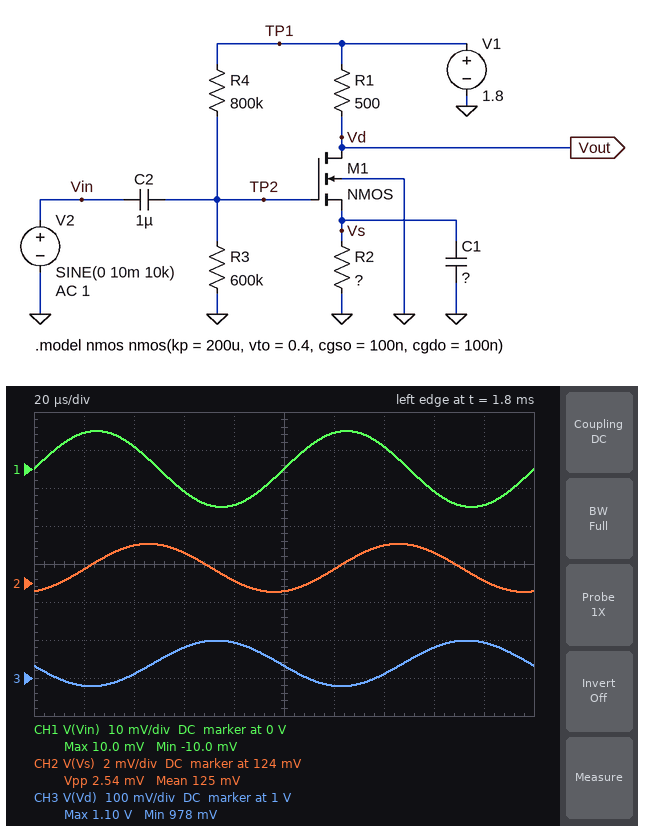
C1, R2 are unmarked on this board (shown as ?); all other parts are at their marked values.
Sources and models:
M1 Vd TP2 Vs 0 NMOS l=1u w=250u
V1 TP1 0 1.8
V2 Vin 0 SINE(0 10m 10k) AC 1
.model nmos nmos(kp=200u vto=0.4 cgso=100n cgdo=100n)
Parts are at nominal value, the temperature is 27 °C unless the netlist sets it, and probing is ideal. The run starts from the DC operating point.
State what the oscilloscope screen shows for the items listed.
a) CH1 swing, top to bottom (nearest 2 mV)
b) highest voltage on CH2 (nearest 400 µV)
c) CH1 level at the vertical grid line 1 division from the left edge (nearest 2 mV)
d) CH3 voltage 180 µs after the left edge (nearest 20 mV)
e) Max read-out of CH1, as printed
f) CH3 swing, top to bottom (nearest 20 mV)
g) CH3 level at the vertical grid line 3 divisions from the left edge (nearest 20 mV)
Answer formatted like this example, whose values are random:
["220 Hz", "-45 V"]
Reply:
["20 mV", "126.0 mV", "10 mV", "1.10 V", "10.0 mV", "120 mV", "1.08 V"]
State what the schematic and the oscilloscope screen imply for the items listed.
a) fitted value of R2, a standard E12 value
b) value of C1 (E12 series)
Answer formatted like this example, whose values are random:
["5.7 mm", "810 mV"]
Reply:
["82 Ω", "1.5 µF"]
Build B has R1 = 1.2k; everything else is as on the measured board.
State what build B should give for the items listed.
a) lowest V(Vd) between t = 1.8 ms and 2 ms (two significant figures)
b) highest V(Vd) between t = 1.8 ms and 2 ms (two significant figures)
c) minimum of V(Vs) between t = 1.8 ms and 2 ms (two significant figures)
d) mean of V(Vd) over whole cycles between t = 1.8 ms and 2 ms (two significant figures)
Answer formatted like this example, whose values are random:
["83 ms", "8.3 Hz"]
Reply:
["230 mV", "250 mV", "110 mV", "240 mV"]
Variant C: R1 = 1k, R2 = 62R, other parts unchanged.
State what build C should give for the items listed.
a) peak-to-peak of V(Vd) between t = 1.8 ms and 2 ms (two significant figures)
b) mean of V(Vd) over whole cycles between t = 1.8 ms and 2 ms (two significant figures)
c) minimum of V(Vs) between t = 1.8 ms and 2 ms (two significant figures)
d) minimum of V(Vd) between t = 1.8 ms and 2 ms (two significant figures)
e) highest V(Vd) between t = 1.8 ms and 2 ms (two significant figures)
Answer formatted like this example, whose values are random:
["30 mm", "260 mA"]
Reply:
["23 mV", "250 mV", "96 mV", "240 mV", "270 mV"]
